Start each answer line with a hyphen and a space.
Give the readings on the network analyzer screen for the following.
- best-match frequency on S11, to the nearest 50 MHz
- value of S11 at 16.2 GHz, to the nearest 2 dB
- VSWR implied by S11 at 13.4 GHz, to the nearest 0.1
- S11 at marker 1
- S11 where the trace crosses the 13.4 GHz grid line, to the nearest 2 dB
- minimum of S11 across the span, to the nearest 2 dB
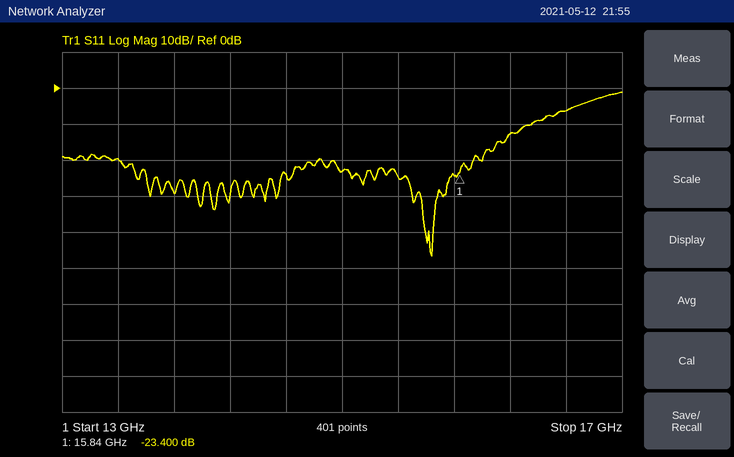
- 15.65 GHz
- -12 dB
- 1.2
- -23.400 dB
- -20 dB
- -46 dB
